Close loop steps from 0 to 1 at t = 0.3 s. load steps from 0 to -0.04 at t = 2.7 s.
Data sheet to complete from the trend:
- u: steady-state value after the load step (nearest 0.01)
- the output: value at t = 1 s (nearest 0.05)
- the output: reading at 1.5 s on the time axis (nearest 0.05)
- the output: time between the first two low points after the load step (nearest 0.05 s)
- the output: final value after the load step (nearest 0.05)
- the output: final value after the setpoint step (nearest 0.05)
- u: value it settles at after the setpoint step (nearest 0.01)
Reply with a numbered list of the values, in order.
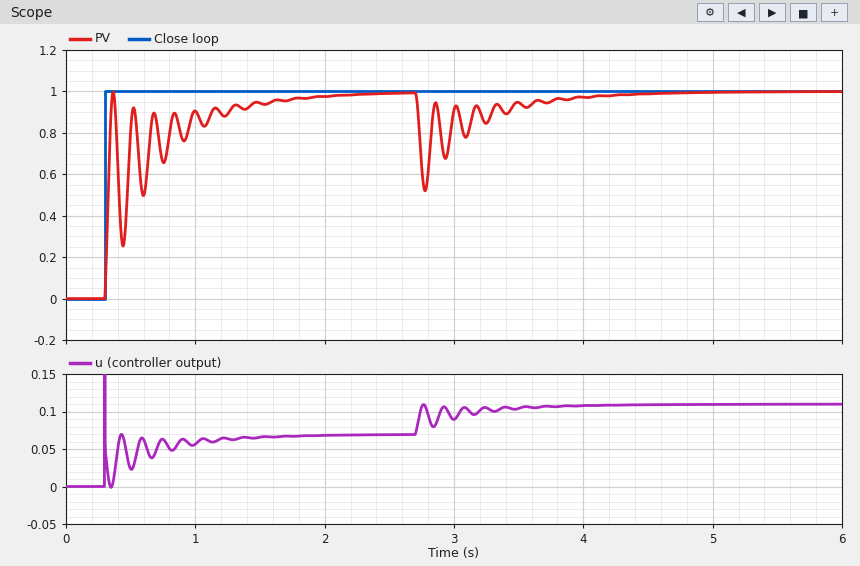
1. 0.11
2. 0.90
3. 0.95
4. 0.15 s
5. 1.00
6. 1.00
7. 0.07
